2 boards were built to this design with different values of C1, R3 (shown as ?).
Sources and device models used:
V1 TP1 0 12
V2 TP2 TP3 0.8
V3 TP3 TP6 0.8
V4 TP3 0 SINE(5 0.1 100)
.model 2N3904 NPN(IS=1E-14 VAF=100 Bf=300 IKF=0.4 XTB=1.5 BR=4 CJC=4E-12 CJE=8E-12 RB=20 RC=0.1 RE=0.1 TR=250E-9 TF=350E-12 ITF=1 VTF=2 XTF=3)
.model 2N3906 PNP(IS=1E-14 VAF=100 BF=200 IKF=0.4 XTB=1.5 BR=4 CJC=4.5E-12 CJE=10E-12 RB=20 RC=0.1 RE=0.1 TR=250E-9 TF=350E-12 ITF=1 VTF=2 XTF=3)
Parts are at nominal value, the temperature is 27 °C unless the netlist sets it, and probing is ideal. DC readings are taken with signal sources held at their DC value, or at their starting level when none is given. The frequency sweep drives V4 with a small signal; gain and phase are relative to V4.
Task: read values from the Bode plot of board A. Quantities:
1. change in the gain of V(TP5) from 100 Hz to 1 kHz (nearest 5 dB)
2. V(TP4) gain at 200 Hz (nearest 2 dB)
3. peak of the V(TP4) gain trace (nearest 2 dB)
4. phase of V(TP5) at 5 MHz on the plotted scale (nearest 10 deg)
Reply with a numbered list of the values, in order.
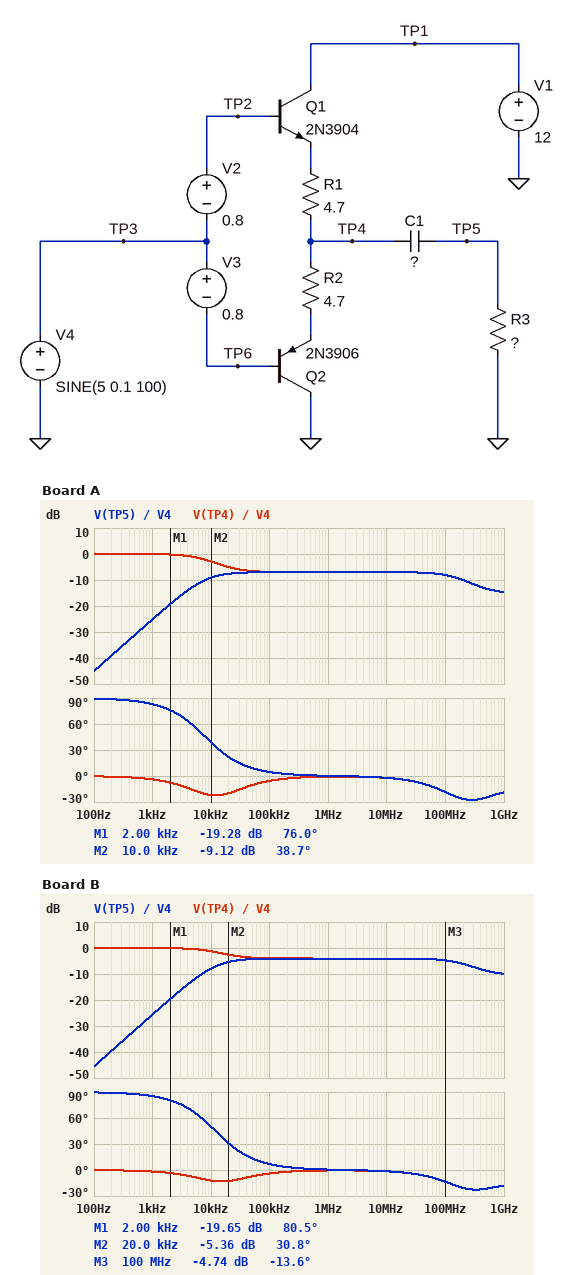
1. 20 dB
2. 0 dB
3. 0 dB
4. 0 deg
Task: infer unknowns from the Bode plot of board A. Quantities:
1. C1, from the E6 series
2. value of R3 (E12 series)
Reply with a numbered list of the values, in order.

1. 3.3 µF
2. 2.7 Ω
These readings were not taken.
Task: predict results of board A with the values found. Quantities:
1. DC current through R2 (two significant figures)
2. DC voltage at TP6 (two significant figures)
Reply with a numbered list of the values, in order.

1. 15 mA
2. 4.2 V
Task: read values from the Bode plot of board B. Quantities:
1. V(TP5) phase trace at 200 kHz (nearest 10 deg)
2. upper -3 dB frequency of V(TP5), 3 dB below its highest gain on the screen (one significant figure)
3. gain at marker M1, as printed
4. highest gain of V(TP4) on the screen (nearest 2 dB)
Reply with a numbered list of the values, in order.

1. 0 deg
2. 300 MHz
3. -19.65 dB
4. 0 dB
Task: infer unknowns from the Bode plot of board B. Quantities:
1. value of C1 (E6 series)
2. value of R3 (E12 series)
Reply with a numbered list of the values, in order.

1. 1.5 µF
2. 5.6 Ω
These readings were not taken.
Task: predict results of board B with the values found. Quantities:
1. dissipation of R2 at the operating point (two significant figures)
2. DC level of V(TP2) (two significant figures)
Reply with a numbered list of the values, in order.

1. 1.1 mW
2. 5.8 V
